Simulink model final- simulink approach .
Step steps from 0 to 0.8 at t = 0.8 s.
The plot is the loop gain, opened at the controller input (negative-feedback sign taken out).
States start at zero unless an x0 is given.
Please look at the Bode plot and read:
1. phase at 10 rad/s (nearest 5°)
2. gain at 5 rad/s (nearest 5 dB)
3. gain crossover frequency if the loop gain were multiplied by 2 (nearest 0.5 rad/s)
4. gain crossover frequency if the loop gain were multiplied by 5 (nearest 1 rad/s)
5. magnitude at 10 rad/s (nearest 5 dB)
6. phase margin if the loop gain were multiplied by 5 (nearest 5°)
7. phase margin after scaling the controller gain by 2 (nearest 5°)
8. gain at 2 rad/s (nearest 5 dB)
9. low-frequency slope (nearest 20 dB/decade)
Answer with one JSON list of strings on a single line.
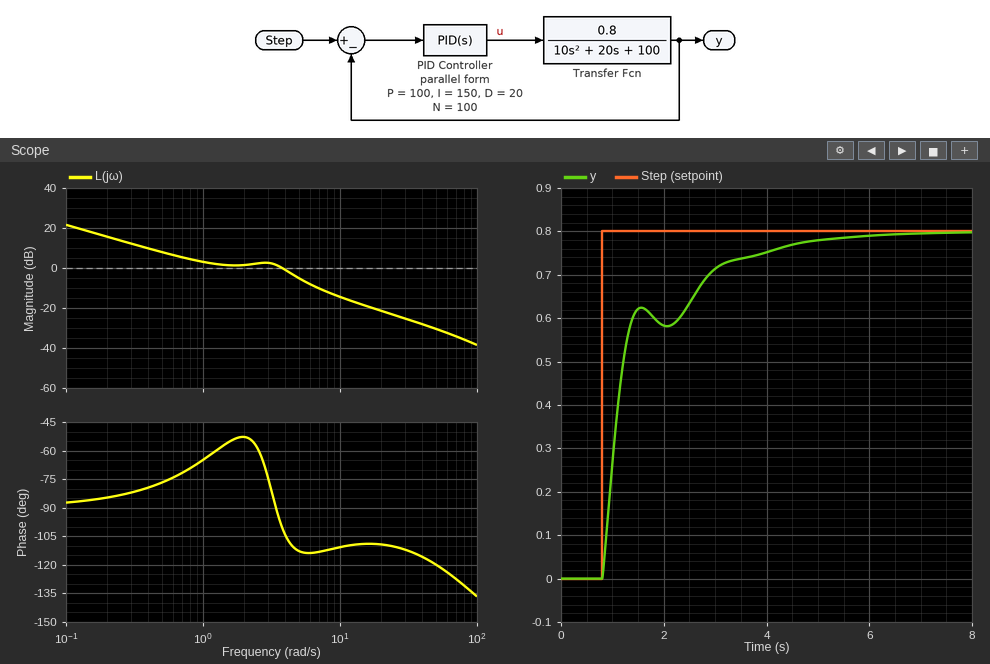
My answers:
["-110°", "-5 dB", "5.5 rad/s", "10 rad/s", "-15 dB", "70°", "65°", "0 dB", "-20 dB/decade"]
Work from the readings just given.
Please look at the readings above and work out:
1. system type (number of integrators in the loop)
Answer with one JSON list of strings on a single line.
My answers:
["1"]
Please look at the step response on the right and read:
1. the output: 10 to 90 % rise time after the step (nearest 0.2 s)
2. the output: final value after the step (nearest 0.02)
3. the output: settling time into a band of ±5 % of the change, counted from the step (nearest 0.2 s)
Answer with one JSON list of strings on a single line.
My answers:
["2.2 s", "0.80", "3.4 s"]
